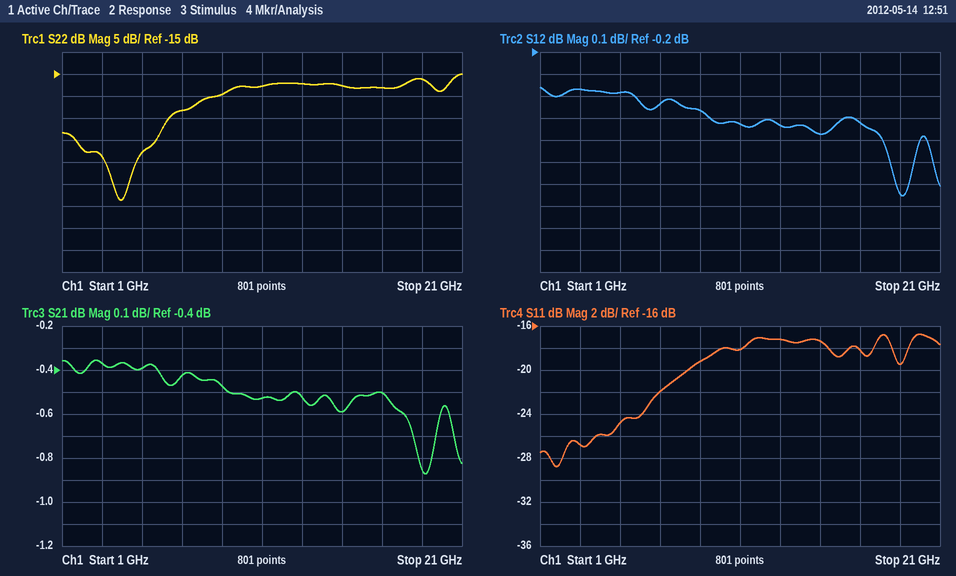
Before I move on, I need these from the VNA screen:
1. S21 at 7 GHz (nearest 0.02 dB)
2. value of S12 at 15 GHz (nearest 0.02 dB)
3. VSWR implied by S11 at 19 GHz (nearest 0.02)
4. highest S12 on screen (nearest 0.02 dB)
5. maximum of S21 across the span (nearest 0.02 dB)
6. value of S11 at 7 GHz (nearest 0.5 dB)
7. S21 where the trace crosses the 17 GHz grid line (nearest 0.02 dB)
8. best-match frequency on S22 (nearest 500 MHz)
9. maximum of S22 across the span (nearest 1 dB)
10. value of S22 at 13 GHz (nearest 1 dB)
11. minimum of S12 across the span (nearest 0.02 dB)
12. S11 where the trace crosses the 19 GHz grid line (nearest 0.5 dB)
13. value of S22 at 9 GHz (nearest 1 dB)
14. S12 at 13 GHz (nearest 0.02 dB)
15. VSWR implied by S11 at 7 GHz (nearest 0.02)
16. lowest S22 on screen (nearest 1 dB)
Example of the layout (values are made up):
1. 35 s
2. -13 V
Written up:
1. -0.42 dB
2. -0.58 dB
3. 1.24
4. -0.36 dB
5. -0.36 dB
6. -22.0 dB
7. -0.50 dB
8. 4.0 GHz
9. -15 dB
10. -17 dB
11. -0.86 dB
12. -19.5 dB
13. -20 dB
14. -0.54 dB
15. 1.18
16. -44 dB
